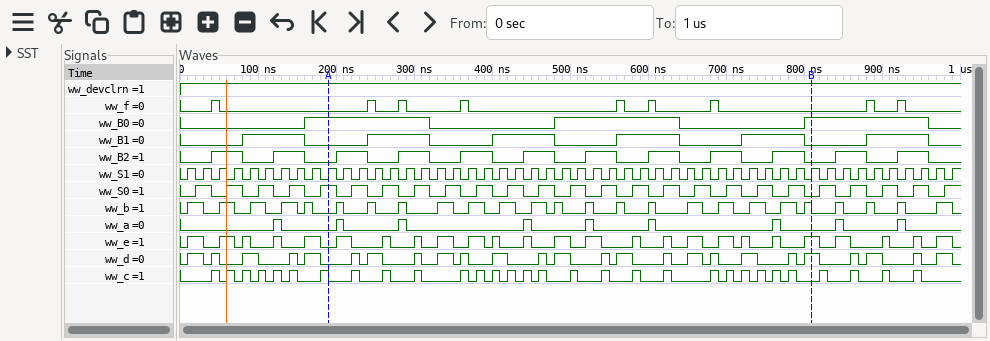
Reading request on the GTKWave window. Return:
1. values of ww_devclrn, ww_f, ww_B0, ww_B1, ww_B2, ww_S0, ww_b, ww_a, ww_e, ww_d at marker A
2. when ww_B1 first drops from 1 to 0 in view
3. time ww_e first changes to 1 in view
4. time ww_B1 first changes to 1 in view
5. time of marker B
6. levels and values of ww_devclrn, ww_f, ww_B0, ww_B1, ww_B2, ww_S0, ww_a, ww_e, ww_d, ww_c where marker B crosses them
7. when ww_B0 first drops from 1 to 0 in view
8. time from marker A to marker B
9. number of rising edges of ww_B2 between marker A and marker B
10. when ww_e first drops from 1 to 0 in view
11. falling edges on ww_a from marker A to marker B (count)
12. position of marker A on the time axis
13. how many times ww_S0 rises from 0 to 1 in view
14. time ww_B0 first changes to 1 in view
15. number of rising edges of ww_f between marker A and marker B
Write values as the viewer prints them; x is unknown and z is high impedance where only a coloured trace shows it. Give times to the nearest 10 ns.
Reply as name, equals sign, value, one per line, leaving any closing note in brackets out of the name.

values of ww_devclrn, ww_f, ww_B0, ww_B1, ww_B2, ww_S0, ww_b, ww_a, ww_e, ww_d at marker A = ww_devclrn=1, ww_f=0, ww_B0=1, ww_B1=0, ww_B2=0, ww_S0=1, ww_b=0, ww_a=0, ww_e=0, ww_d=0
when ww_B1 first drops from 1 to 0 in view = 160 ns
time ww_e first changes to 1 in view = 10 ns
time ww_B1 first changes to 1 in view = 80 ns
time of marker B = 810 ns
levels and values of ww_devclrn, ww_f, ww_B0, ww_B1, ww_B2, ww_S0, ww_a, ww_e, ww_d, ww_c where marker B crosses them = ww_devclrn=1, ww_f=0, ww_B0=1, ww_B1=0, ww_B2=0, ww_S0=0, ww_a=0, ww_e=1, ww_d=1, ww_c=0
when ww_B0 first drops from 1 to 0 in view = 320 ns
time from marker A to marker B = 620 ns
number of rising edges of ww_B2 between marker A and marker B = 8
when ww_e first drops from 1 to 0 in view = 30 ns
falling edges on ww_a from marker A to marker B = 6
position of marker A on the time axis = 190 ns
how many times ww_S0 rises from 0 to 1 in view = 25
time ww_B0 first changes to 1 in view = 160 ns
number of rising edges of ww_f between marker A and marker B = 6
